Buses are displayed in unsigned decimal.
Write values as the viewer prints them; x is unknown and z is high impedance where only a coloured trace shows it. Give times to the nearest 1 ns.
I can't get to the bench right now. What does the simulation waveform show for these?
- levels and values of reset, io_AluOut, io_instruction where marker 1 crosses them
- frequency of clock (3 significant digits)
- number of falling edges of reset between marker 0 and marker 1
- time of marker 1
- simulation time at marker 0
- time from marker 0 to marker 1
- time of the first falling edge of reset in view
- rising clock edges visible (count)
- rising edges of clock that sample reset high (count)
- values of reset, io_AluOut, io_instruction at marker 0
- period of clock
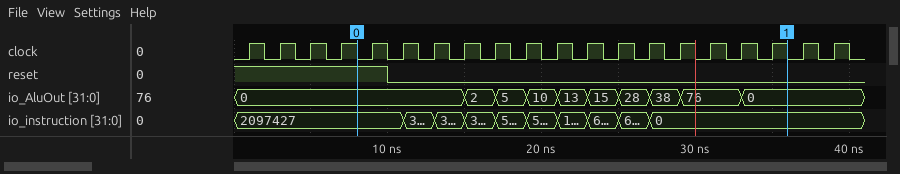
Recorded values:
reset=0, io_AluOut=0, io_instruction=0
500 MHz
1
36 ns
8 ns
28 ns
10 ns
20
5
reset=1, io_AluOut=0, io_instruction=2097427
2 ns
